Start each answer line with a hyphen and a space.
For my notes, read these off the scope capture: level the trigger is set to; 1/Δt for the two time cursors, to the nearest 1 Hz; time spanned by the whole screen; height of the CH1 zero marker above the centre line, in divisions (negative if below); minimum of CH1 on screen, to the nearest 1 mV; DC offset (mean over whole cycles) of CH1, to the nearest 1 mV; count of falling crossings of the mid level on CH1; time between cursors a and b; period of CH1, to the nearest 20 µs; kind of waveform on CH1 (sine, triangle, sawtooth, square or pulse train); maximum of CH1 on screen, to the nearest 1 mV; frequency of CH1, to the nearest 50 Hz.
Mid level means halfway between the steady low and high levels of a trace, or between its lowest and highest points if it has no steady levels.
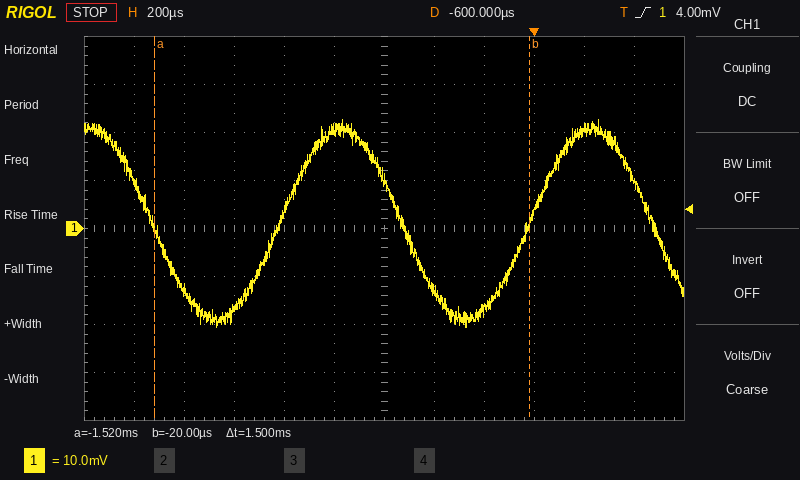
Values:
- 4.00 mV
- 667 Hz
- 2.4 ms
- 0.0 div
- -21 mV
- 1 mV
- 3
- 1.5 ms
- 1.00 ms
- sine
- 23 mV
- 1.00 kHz
